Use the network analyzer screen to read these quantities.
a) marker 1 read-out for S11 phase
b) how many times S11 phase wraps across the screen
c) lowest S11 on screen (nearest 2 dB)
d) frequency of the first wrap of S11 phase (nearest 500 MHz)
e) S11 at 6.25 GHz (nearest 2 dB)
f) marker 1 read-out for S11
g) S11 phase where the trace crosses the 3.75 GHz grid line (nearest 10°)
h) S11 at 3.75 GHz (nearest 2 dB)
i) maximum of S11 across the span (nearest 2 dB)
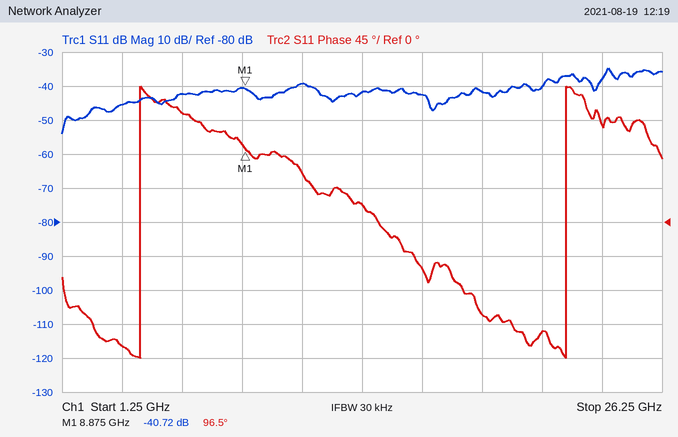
96.5°
2
-54 dB
4.5 GHz
-42 dB
-40.72 dB
-160°
-46 dB
-34 dB
